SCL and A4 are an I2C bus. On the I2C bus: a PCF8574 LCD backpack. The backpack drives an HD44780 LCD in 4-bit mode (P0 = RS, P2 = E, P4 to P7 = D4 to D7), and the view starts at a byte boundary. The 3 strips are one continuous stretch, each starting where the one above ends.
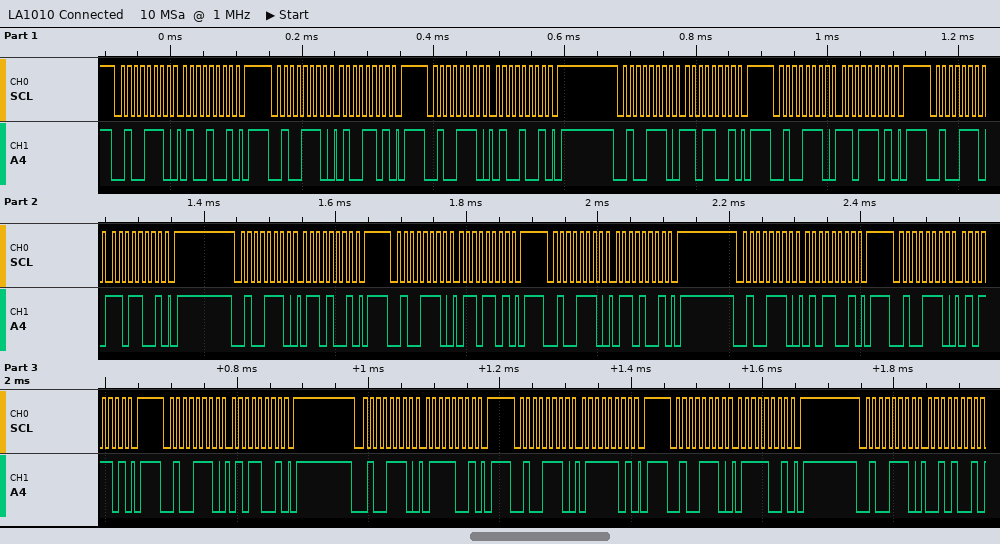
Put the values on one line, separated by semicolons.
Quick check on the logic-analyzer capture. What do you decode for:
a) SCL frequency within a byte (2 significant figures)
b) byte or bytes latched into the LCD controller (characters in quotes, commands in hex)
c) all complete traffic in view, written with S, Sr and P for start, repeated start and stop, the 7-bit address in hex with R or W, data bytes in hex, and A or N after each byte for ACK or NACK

100 kHz; 'M' 'e'; S 27W A 49 A P S 27W A 4D A P S 27W A 49 A P S 27W A D9 A P S 27W A DD A P S 27W A D9 A P S 27W A 69 A P S 27W A 6D A P S 27W A 69 A P S 27W A 59 A P S 27W A 5D A P S 27W A 59 A P S 27W A 79 A P S 27W A 7D A P S 27W A 79 A P S 27W A 29 A
